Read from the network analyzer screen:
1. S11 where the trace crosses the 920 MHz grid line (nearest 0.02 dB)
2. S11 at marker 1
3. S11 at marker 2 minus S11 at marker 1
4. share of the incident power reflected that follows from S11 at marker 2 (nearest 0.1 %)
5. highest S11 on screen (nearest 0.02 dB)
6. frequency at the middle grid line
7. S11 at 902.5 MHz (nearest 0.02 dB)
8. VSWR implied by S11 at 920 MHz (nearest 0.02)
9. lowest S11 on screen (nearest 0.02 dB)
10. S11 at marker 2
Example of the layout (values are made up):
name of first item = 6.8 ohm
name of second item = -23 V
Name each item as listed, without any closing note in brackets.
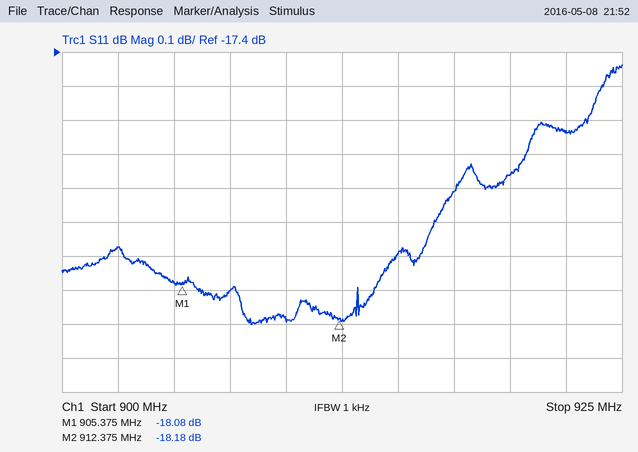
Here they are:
S11 where the trace crosses the 920 MHz grid line = -17.76 dB
S11 at marker 1 = -18.08 dB
S11 at marker 2 minus S11 at marker 1 = -0.10 dB
share of the incident power reflected that follows from S11 at marker 2 = 1.5 %
highest S11 on screen = -17.44 dB
frequency at the middle grid line = 912.5 MHz
S11 at 902.5 MHz = -17.98 dB
VSWR implied by S11 at 920 MHz = 1.30
lowest S11 on screen = -18.20 dB
S11 at marker 2 = -18.18 dB
